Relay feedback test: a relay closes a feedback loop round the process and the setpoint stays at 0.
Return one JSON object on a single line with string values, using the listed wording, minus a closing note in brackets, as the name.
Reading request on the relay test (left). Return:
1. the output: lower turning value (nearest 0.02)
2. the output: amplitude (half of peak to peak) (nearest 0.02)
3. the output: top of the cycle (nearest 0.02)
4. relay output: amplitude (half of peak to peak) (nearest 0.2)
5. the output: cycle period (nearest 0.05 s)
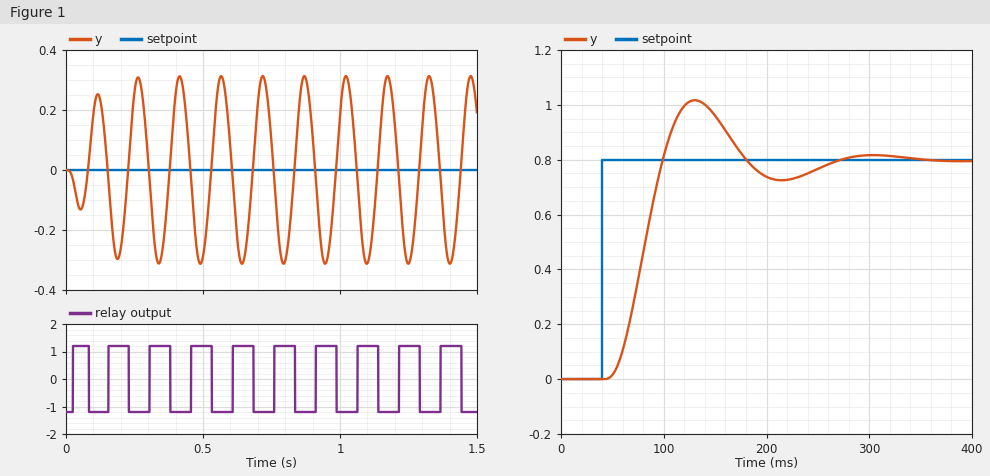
{"the output: lower turning value": "-0.32", "the output: amplitude (half of peak to peak)": "0.32", "the output: top of the cycle": "0.32", "relay output: amplitude (half of peak to peak)": "1.2", "the output: cycle period": "0.15 s"}
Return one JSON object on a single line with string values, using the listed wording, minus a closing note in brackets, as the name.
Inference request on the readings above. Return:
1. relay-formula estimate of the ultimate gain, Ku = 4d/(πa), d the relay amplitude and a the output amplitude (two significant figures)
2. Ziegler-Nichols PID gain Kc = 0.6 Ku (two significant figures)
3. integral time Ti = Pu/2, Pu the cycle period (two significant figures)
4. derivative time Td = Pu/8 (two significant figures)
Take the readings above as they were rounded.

{"relay-formula estimate of the ultimate gain, Ku = 4d/(πa), d the relay amplitude and a the output amplitude": "4.8", "Ziegler-Nichols PID gain Kc = 0.6 Ku": "2.9", "integral time Ti = Pu/2, Pu the cycle period": "0.075 s", "derivative time Td = Pu/8": "0.019 s"}
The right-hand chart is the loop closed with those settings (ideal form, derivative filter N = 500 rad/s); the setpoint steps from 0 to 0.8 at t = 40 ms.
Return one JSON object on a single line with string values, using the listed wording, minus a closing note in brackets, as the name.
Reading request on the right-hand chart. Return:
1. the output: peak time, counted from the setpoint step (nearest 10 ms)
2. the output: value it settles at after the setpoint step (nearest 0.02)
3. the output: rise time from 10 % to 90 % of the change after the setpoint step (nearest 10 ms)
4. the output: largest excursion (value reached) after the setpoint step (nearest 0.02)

{"the output: peak time, counted from the setpoint step": "90 ms", "the output: value it settles at after the setpoint step": "0.80", "the output: rise time from 10 % to 90 % of the change after the setpoint step": "40 ms", "the output: largest excursion (value reached) after the setpoint step": "1.02"}
